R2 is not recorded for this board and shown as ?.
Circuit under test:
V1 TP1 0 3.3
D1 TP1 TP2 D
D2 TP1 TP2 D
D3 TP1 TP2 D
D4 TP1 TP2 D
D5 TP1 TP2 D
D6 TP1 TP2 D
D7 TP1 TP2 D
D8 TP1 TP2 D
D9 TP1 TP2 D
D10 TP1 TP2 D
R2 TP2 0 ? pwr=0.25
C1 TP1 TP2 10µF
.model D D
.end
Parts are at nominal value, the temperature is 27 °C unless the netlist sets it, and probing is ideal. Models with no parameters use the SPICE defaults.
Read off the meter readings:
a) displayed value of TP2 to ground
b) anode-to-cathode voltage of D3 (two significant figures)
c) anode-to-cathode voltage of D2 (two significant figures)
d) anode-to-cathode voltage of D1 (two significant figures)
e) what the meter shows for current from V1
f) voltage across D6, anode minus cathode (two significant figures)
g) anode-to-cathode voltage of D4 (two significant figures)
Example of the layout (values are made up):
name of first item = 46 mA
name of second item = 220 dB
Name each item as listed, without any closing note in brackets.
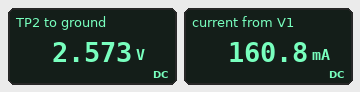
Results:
displayed value of TP2 to ground = 2.573 V
anode-to-cathode voltage of D3 = 730 mV
anode-to-cathode voltage of D2 = 730 mV
anode-to-cathode voltage of D1 = 730 mV
what the meter shows for current from V1 = 160.8 mA
voltage across D6, anode minus cathode = 730 mV
anode-to-cathode voltage of D4 = 730 mV
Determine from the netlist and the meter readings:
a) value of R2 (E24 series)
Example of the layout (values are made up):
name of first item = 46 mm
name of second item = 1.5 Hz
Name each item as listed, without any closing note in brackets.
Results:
value of R2 = 16 Ω
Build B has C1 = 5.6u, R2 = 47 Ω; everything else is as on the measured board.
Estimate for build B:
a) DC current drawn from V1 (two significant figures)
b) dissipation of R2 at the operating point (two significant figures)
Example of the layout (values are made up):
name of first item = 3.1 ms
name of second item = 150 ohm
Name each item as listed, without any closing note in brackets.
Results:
DC current drawn from V1 = 55 mA
dissipation of R2 at the operating point = 140 mW
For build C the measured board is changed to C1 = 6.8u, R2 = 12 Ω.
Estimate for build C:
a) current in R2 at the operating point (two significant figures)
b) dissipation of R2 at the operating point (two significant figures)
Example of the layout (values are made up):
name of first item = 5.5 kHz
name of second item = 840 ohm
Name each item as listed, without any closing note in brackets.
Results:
current in R2 at the operating point = 210 mA
dissipation of R2 at the operating point = 550 mW
